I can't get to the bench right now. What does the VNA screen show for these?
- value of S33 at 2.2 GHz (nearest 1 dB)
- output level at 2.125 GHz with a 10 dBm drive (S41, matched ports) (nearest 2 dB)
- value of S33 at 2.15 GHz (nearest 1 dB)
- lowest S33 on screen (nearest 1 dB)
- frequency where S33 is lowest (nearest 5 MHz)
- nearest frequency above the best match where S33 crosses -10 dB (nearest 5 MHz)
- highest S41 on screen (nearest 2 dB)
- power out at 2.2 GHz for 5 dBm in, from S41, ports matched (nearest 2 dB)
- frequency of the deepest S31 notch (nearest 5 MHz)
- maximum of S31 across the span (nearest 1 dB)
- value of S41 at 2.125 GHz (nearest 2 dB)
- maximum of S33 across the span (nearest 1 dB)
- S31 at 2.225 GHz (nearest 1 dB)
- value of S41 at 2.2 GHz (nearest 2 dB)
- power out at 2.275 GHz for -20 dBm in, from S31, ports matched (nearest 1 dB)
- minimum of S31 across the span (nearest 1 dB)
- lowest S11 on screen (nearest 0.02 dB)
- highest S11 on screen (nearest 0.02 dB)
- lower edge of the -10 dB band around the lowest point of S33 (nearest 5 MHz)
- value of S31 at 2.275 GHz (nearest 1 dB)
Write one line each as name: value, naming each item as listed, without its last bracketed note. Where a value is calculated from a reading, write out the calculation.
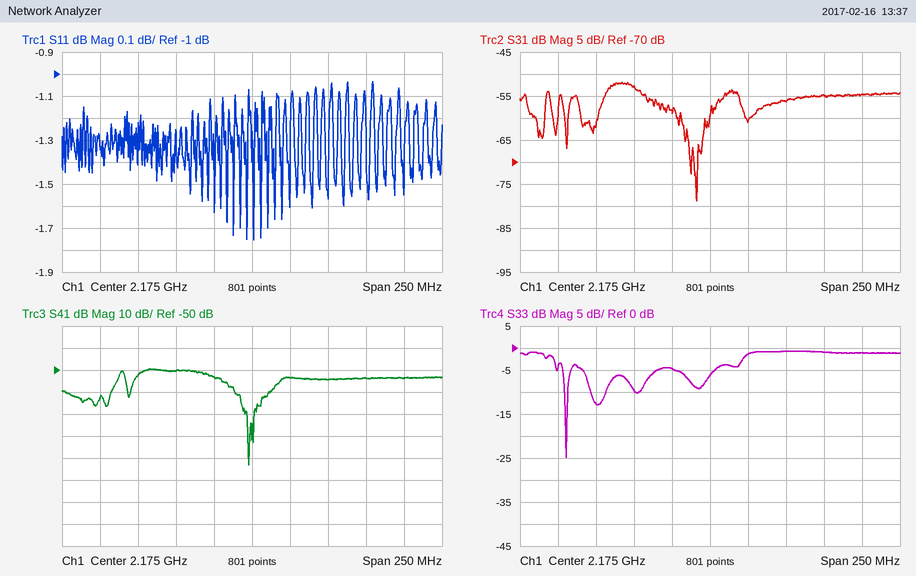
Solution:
value of S33 at 2.2 GHz: -1 dB
output level at 2.125 GHz with a 10 dBm drive (S41, matched ports): 10 dBm + (-50 dB) = -40 dBm
value of S33 at 2.15 GHz: -5 dB
lowest S33 on screen: -25 dB
frequency where S33 is lowest: 2.080 GHz
nearest frequency above the best match where S33 crosses -10 dB: 2.080 GHz
highest S41 on screen: -50 dB
power out at 2.2 GHz for 5 dBm in, from S41, ports matched: 5 dBm + (-54 dB) = -48 dBm
frequency of the deepest S31 notch: 2.165 GHz
maximum of S31 across the span: -52 dB
value of S41 at 2.125 GHz: -50 dB
maximum of S33 across the span: -1 dB
S31 at 2.225 GHz: -56 dB
value of S41 at 2.2 GHz: -54 dB
power out at 2.275 GHz for -20 dBm in, from S31, ports matched: -20 dBm + (-55 dB) = -75 dBm
minimum of S31 across the span: -79 dB
lowest S11 on screen: -1.76 dB
highest S11 on screen: -1.04 dB
lower edge of the -10 dB band around the lowest point of S33: 2.080 GHz
value of S31 at 2.275 GHz: -55 dB
